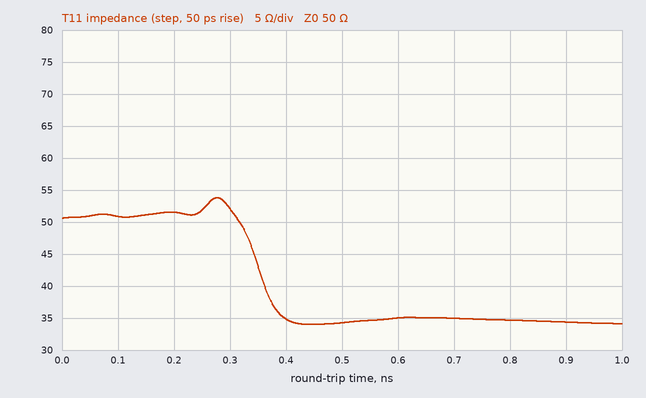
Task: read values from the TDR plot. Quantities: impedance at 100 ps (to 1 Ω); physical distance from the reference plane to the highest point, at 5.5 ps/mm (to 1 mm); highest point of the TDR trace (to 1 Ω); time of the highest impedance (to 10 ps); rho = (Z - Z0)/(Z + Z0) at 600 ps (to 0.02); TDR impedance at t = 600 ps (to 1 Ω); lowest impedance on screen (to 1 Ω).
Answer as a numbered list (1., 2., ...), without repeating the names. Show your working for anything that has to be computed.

1. 51 Ω
2. 280 ps / 2 / 5.5 ps/mm ≈ 25 mm
3. 54 Ω
4. 280 ps
5. (35 − 50)/(35 + 50) ≈ -0.18
6. 35 Ω
7. 34 Ω
